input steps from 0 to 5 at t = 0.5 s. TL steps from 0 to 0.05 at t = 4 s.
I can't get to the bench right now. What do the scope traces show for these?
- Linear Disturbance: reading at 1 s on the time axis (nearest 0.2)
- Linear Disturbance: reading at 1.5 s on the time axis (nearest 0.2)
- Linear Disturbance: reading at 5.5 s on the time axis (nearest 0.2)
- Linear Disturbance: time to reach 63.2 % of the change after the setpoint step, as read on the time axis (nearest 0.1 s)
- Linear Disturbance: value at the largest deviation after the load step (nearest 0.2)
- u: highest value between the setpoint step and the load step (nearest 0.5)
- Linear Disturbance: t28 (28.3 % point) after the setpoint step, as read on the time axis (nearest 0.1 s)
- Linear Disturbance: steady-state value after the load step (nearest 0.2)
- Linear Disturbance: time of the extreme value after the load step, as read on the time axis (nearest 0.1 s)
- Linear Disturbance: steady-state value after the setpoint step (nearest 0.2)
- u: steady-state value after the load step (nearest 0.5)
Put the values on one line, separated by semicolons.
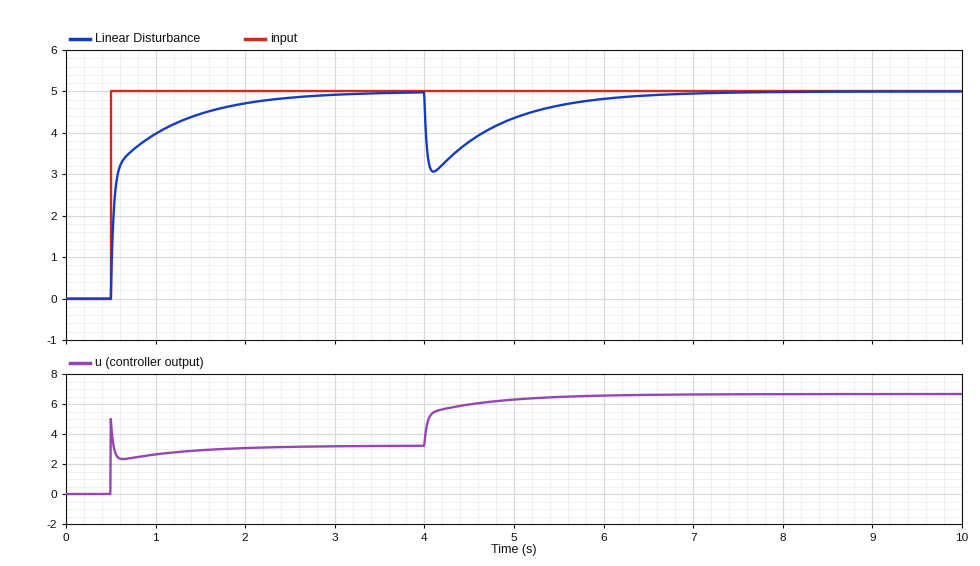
4.0; 4.4; 4.6; 0.6 s; 3.0; 5.0; 0.5 s; 5.0; 4.1 s; 5.0; 6.5
